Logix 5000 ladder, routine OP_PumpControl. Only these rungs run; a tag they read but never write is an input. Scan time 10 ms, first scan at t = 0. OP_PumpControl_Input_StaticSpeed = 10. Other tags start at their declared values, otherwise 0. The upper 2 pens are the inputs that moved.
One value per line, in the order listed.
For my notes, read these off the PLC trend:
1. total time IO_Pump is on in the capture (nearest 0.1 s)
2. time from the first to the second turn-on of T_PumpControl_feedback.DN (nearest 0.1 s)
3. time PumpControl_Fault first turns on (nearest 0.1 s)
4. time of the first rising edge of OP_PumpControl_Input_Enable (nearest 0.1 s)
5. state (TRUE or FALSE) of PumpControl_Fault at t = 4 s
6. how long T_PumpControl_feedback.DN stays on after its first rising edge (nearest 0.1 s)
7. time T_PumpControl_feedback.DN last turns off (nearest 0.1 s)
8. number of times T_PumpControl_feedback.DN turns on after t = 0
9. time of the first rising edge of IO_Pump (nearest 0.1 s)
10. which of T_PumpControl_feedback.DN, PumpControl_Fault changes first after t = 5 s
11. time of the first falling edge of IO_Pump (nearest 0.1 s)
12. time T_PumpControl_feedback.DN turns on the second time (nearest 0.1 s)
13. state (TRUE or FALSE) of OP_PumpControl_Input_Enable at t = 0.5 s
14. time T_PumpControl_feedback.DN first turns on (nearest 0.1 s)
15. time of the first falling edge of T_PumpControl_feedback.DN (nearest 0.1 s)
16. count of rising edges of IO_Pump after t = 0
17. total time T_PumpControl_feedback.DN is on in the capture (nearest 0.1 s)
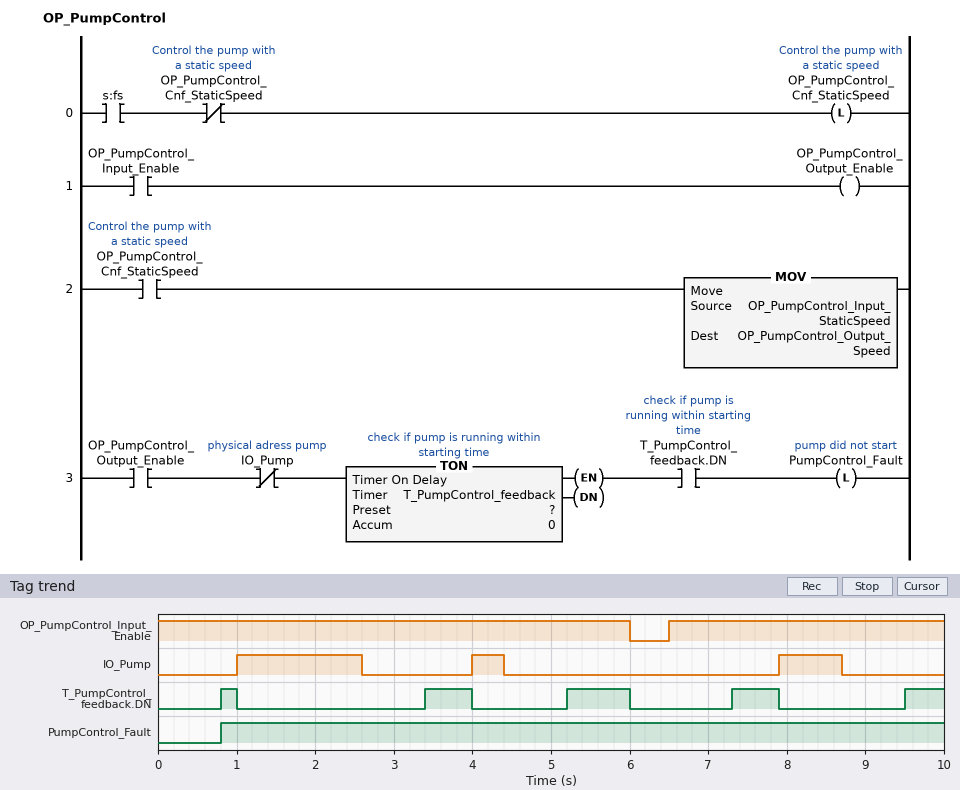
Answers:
2.8 s
2.6 s
0.8 s
6.5 s
TRUE
0.2 s
7.9 s
5
1.0 s
T_PumpControl_feedback.DN
2.6 s
3.4 s
TRUE
0.8 s
1.0 s
3
2.7 s
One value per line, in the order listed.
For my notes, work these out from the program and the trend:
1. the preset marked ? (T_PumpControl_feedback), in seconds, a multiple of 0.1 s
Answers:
0.8 s
